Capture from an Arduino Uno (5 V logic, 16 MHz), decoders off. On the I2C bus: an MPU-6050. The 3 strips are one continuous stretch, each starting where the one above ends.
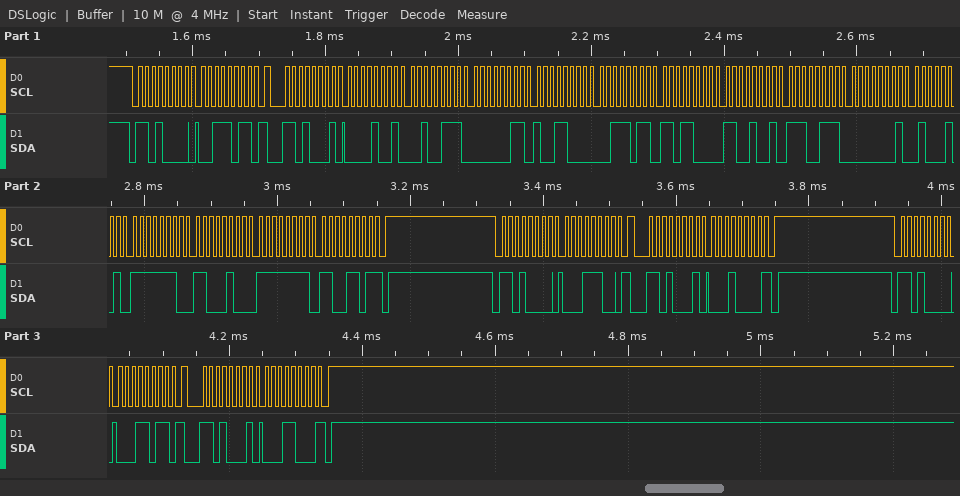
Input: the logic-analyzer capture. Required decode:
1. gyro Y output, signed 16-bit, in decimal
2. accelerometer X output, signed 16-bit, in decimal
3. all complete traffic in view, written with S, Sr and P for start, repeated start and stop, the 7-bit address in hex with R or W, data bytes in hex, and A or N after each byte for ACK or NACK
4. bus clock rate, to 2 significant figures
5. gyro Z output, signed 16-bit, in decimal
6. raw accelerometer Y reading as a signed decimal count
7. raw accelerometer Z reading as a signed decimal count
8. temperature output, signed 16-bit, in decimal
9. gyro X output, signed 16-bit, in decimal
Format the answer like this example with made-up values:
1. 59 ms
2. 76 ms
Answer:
1. -316
2. 2343
3. S 68W A 3B A Sr 68R A 09 A 27 A 03 A 98 A 3B A D8 A C9 A E7 A 01 A 45 A FE A C4 A FF A CD N P S 68W A 1C A Sr 68R A 10 N P S 68W A 1B A Sr 68R A 18 N P
4. 100 kHz
5. -51
6. 920
7. 15320
8. -13849
9. 325
